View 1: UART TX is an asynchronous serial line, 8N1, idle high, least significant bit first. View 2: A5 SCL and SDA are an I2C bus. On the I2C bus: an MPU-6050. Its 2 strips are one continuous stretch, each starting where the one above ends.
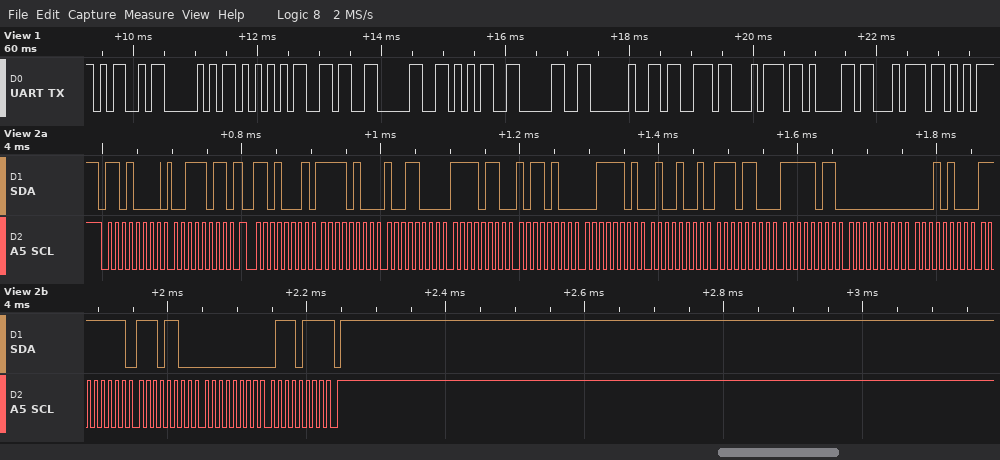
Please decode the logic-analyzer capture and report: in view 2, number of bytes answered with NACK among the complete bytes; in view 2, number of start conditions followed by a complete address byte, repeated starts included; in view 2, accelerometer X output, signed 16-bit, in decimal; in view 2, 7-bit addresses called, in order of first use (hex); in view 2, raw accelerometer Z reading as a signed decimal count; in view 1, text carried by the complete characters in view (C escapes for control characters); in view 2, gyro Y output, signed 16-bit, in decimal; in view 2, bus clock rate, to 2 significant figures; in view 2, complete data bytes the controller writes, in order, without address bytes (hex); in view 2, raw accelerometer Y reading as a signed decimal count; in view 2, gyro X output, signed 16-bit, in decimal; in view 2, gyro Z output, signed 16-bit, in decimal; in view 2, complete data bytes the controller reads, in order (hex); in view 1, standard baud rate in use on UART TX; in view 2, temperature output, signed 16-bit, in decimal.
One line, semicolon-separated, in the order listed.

1; 2; -2920; 0x68; 15689; "MPU6050 stat"; -20; 100 kHz; 3B; -2380; 20; 119; F4 98 F6 B4 3D 49 EC FB 00 14 FF EC 00 77; 9600 baud; -4869
